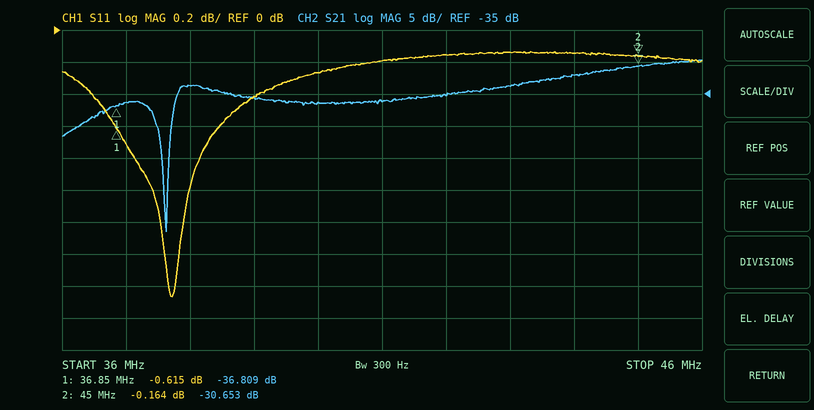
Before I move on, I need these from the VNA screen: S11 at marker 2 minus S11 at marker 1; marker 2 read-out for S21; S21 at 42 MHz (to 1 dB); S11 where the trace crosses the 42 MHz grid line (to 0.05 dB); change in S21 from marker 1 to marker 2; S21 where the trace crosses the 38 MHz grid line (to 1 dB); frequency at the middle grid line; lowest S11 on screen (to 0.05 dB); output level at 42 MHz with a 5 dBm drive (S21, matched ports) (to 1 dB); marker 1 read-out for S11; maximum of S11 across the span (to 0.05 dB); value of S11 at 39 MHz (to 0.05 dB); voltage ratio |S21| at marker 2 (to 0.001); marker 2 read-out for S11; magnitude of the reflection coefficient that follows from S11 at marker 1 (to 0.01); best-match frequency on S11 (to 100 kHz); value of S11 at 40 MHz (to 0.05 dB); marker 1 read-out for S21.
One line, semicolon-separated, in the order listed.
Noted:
0.451 dB; -30.653 dB; -35 dB; -0.15 dB; 6.156 dB; -34 dB; 41 MHz; -1.65 dB; -30 dBm; -0.615 dB; -0.15 dB; -0.40 dB; 0.029; -0.164 dB; 0.93; 37.7 MHz; -0.25 dB; -36.809 dB
